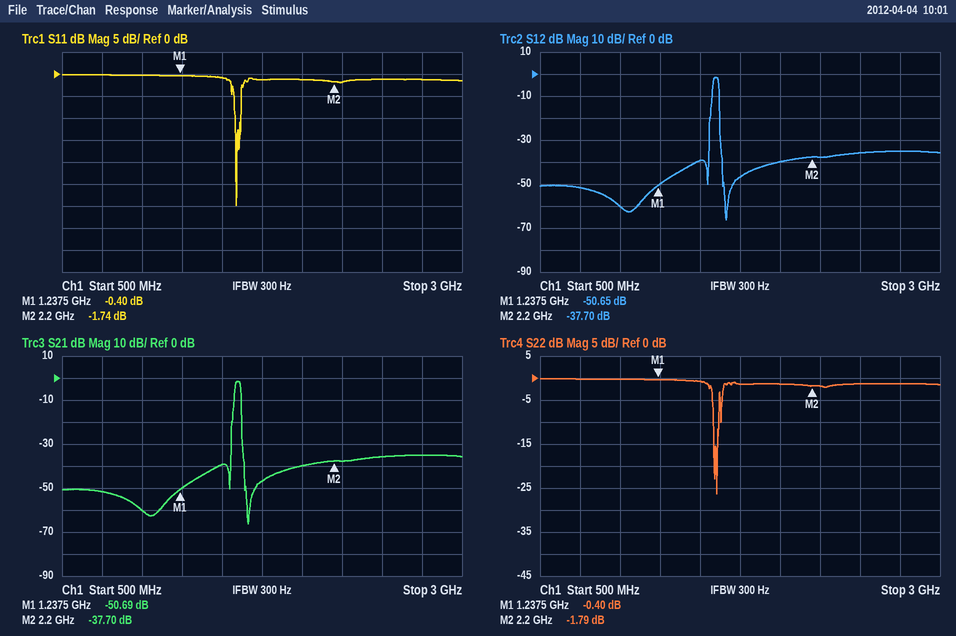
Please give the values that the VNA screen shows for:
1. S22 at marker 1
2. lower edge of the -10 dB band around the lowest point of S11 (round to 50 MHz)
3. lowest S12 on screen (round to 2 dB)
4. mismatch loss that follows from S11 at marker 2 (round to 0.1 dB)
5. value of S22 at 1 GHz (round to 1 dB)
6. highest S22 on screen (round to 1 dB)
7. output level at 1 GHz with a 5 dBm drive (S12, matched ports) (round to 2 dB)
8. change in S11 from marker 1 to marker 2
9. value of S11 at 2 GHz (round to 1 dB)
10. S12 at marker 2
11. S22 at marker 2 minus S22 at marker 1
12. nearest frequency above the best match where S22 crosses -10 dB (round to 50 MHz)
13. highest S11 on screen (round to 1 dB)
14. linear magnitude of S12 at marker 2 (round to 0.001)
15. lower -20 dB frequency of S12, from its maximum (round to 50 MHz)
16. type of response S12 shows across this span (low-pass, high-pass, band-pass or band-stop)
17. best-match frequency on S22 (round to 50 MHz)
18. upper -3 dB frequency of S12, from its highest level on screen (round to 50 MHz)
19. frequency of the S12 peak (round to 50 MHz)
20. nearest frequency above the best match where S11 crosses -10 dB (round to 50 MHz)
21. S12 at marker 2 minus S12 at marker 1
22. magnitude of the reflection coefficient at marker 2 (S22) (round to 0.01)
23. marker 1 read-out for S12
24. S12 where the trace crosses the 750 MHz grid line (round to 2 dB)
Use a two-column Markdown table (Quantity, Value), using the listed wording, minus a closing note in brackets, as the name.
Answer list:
| Quantity | Value |
|---|---|
| S22 at marker 1 | -0.40 dB |
| lower edge of the -10 dB band around the lowest point of S11 | 1.60 GHz |
| lowest S12 on screen | -66 dB |
| mismatch loss that follows from S11 at marker 2 | 4.8 dB |
| value of S22 at 1 GHz | 0 dB |
| highest S22 on screen | 0 dB |
| output level at 1 GHz with a 5 dBm drive (S12, matched ports) | -56 dBm |
| change in S11 from marker 1 to marker 2 | -1.34 dB |
| value of S11 at 2 GHz | -1 dB |
| S12 at marker 2 | -37.70 dB |
| S22 at marker 2 minus S22 at marker 1 | -1.39 dB |
| nearest frequency above the best match where S22 crosses -10 dB | 1.60 GHz |
| highest S11 on screen | 0 dB |
| linear magnitude of S12 at marker 2 | 0.013 |
| lower -20 dB frequency of S12, from its maximum | 1.55 GHz |
| type of response S12 shows across this span | band-pass |
| best-match frequency on S22 | 1.60 GHz |
| upper -3 dB frequency of S12, from its highest level on screen | 1.60 GHz |
| frequency of the S12 peak | 1.60 GHz |
| nearest frequency above the best match where S11 crosses -10 dB | 1.60 GHz |
| S12 at marker 2 minus S12 at marker 1 | 12.95 dB |
| magnitude of the reflection coefficient at marker 2 (S22) | 0.81 |
| marker 1 read-out for S12 | -50.65 dB |
| S12 where the trace crosses the 750 MHz grid line | -52 dB |
